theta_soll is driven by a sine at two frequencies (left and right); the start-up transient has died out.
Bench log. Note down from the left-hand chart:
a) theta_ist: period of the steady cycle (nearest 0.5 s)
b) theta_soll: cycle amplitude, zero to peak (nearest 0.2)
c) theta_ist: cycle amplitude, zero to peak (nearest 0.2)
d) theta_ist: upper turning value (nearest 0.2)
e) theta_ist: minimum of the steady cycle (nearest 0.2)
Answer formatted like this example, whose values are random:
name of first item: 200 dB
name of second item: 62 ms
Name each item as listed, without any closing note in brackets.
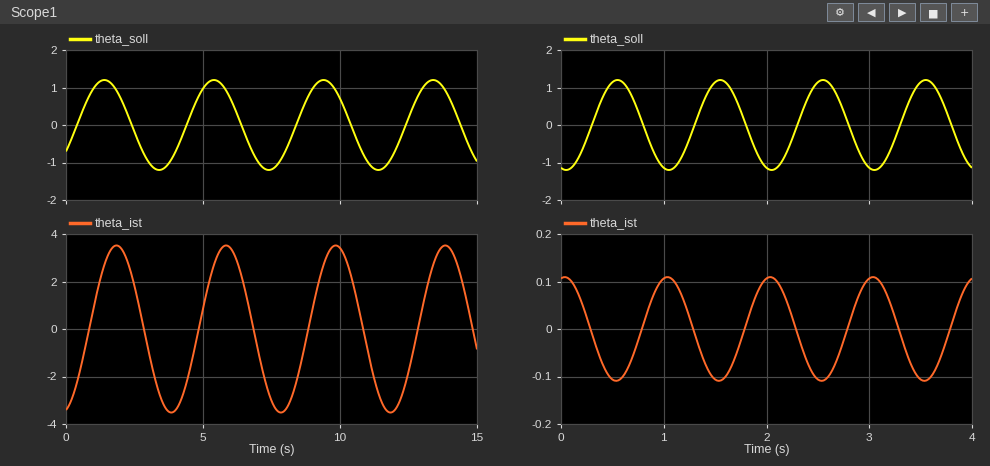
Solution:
theta_ist: period of the steady cycle: 4.0 s
theta_soll: cycle amplitude, zero to peak: 1.2
theta_ist: cycle amplitude, zero to peak: 3.6
theta_ist: upper turning value: 3.6
theta_ist: minimum of the steady cycle: -3.6
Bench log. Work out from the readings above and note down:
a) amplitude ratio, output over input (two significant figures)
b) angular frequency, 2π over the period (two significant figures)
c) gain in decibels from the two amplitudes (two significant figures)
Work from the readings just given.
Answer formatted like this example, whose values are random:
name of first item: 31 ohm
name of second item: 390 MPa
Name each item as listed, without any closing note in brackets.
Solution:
amplitude ratio, output over input: 3.0
angular frequency, 2π over the period: 1.6 rad/s
gain in decibels from the two amplitudes: 9.5 dB
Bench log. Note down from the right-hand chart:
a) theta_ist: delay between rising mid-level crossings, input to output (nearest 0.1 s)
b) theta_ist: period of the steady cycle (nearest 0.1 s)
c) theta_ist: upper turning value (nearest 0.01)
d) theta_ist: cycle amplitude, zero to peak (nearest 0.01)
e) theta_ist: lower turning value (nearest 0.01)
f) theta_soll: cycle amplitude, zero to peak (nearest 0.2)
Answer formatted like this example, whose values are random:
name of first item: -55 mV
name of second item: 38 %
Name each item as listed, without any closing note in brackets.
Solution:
theta_ist: delay between rising mid-level crossings, input to output: 0.5 s
theta_ist: period of the steady cycle: 1.0 s
theta_ist: upper turning value: 0.11
theta_ist: cycle amplitude, zero to peak: 0.11
theta_ist: lower turning value: -0.11
theta_soll: cycle amplitude, zero to peak: 1.2
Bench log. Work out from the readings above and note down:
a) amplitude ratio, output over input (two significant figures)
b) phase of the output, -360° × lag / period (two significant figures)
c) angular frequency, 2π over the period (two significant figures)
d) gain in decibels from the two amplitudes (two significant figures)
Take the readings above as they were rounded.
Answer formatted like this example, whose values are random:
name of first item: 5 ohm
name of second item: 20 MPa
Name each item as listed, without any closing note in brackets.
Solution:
amplitude ratio, output over input: 0.092
phase of the output, -360° × lag / period: -180°
angular frequency, 2π over the period: 6.3 rad/s
gain in decibels from the two amplitudes: -21 dB
